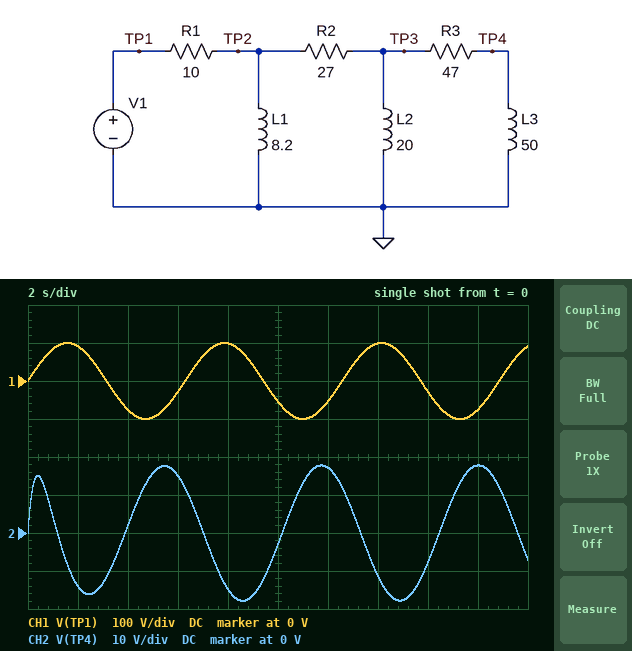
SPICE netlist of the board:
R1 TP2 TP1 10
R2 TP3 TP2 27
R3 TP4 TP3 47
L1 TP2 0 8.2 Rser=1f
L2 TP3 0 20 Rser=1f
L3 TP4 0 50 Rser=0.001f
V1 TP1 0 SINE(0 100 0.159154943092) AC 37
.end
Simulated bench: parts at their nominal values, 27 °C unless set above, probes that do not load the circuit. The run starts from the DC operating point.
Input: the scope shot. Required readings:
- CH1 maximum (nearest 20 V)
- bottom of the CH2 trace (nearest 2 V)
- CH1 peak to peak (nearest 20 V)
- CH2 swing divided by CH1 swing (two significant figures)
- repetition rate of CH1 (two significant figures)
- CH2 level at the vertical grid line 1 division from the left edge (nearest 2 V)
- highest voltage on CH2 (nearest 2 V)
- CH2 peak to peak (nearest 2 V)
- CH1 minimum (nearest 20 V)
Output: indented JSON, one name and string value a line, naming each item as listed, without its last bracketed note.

{
  "CH1 maximum": "100 V",
  "bottom of the CH2 trace": "-18 V",
  "CH1 peak to peak": "200 V",
  "CH2 swing divided by CH1 swing": "0.18",
  "repetition rate of CH1": "160 mHz",
  "CH2 level at the vertical grid line 1 division from the left edge": "-14 V",
  "highest voltage on CH2": "18 V",
  "CH2 peak to peak": "36 V",
  "CH1 minimum": "-100 V"
}
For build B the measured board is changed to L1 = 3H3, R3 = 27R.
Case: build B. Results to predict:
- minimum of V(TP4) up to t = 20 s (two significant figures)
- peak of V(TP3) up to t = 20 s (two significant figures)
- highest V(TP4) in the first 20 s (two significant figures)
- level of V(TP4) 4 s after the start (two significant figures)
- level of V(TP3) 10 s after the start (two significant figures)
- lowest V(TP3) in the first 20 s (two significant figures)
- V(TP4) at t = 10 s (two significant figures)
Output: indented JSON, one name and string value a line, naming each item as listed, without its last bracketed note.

{
  "minimum of V(TP4) up to t = 20 s": "-11 V",
  "peak of V(TP3) up to t = 20 s": "14 V",
  "highest V(TP4) in the first 20 s": "12 V",
  "level of V(TP4) 4 s after the start": "1.1 V",
  "level of V(TP3) 10 s after the start": "-8.0 V",
  "lowest V(TP3) in the first 20 s": "-13 V",
  "V(TP4) at t = 10 s": "-2.1 V"
}
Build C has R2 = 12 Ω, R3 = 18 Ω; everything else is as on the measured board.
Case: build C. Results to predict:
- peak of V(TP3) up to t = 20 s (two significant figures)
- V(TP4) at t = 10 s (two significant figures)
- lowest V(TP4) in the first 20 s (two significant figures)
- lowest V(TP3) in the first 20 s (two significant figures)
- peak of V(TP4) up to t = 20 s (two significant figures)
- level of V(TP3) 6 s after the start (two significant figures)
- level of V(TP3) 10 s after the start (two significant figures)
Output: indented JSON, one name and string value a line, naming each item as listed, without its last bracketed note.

{
  "peak of V(TP3) up to t = 20 s": "34 V",
  "V(TP4) at t = 10 s": "-22 V",
  "lowest V(TP4) in the first 20 s": "-32 V",
  "lowest V(TP3) in the first 20 s": "-34 V",
  "peak of V(TP4) up to t = 20 s": "32 V",
  "level of V(TP3) 6 s after the start": "31 V",
  "level of V(TP3) 10 s after the start": "-30 V"
}
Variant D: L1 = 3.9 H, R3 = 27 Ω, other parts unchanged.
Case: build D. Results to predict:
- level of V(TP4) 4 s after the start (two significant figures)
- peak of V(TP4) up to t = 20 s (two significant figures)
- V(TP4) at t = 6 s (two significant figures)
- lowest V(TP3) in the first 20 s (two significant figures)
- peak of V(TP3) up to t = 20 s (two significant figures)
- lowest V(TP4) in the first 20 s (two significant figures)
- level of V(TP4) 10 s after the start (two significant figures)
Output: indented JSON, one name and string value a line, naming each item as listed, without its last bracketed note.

{
  "level of V(TP4) 4 s after the start": "1.1 V",
  "peak of V(TP4) up to t = 20 s": "13 V",
  "V(TP4) at t = 6 s": "11 V",
  "lowest V(TP3) in the first 20 s": "-14 V",
  "peak of V(TP3) up to t = 20 s": "15 V",
  "lowest V(TP4) in the first 20 s": "-13 V",
  "level of V(TP4) 10 s after the start": "-2.5 V"
}
